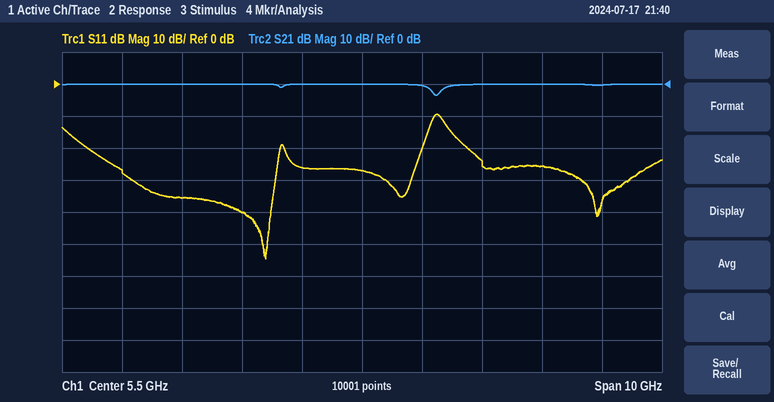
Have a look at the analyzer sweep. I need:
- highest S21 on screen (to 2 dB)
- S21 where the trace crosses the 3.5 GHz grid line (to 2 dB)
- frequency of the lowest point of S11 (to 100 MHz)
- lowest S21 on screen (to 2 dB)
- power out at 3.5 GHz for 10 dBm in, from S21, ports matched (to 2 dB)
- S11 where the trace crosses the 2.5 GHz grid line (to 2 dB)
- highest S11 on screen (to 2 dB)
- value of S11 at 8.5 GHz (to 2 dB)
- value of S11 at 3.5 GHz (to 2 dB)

0 dB
0 dB
3.9 GHz
-4 dB
10 dBm
-36 dB
-10 dB
-26 dB
-40 dB
